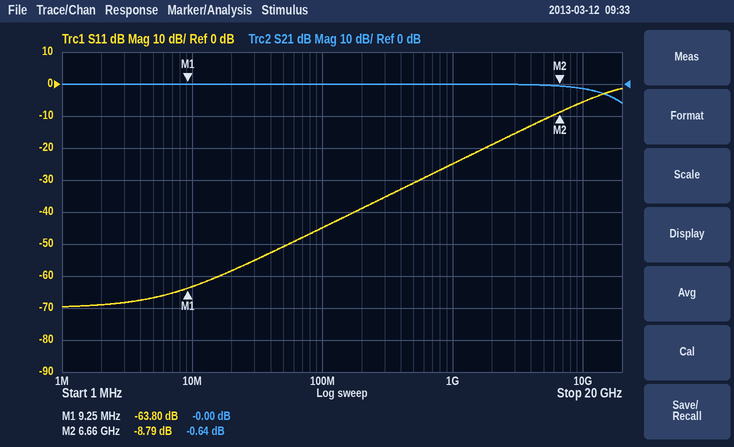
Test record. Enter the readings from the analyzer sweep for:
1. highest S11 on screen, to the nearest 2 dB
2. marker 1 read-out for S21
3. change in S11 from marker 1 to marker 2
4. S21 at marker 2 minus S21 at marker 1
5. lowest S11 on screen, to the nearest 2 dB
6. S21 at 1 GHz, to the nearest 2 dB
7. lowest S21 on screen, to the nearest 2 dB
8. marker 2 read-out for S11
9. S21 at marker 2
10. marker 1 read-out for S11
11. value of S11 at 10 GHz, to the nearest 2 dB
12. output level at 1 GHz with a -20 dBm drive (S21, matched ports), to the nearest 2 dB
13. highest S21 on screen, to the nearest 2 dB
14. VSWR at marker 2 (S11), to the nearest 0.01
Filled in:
-2 dB
-0.00 dB
55.01 dB
-0.64 dB
-70 dB
0 dB
-6 dB
-8.79 dB
-0.64 dB
-63.80 dB
-6 dB
-20 dBm
0 dB
2.14
